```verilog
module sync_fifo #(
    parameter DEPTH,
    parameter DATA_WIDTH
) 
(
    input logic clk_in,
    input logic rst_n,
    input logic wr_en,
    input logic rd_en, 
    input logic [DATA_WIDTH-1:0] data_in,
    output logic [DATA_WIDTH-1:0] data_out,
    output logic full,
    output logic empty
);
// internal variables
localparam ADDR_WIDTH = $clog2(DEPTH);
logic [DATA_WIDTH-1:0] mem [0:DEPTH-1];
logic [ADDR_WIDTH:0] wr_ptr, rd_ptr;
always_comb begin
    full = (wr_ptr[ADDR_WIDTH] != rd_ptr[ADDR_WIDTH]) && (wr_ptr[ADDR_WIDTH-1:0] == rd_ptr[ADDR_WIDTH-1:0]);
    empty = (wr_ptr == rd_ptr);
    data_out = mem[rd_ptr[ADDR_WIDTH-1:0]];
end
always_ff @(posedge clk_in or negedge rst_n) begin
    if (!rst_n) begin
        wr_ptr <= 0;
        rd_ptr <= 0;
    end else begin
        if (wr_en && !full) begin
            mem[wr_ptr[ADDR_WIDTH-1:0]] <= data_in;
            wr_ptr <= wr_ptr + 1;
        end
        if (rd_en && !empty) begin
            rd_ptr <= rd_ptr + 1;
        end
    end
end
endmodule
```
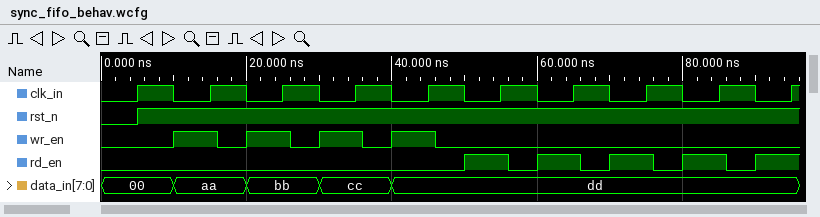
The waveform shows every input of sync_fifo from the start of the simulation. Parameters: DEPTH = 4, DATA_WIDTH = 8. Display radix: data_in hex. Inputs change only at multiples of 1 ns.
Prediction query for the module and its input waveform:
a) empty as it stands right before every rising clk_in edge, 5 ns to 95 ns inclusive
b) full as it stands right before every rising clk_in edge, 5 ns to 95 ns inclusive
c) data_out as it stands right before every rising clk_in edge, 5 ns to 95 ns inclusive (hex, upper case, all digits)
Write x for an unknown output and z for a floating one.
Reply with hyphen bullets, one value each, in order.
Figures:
- 1 1 0 0 0 0 0 0 0 1
- 0 0 0 0 0 1 0 0 0 0
- x, x, AA, AA, AA, AA, BB, CC, DD, AA
